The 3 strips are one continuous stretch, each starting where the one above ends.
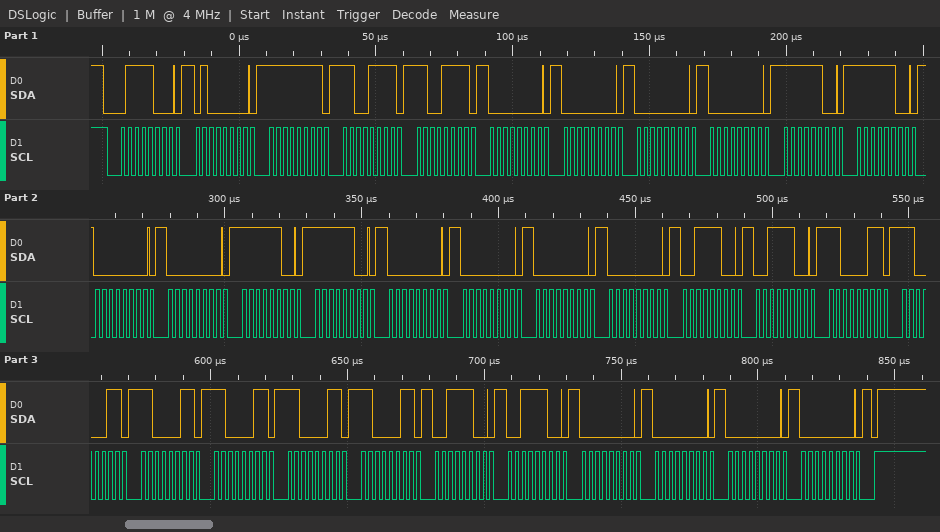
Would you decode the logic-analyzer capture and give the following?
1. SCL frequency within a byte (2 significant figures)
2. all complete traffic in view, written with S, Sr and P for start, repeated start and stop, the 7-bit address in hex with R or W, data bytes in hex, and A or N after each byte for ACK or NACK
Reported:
400 kHz
S 3CW A 40 A FF A CF A CF A 00 A 00 A 00 A 00 A FC A FC A 00 A 00 A FC A FC A 00 A 00 A 00 A 00 A 3C A 3C A C3 A C3 A C3 A C3 A C3 A C3 A 3C A 3C A 00 A 00 A 00 A 00 A P
